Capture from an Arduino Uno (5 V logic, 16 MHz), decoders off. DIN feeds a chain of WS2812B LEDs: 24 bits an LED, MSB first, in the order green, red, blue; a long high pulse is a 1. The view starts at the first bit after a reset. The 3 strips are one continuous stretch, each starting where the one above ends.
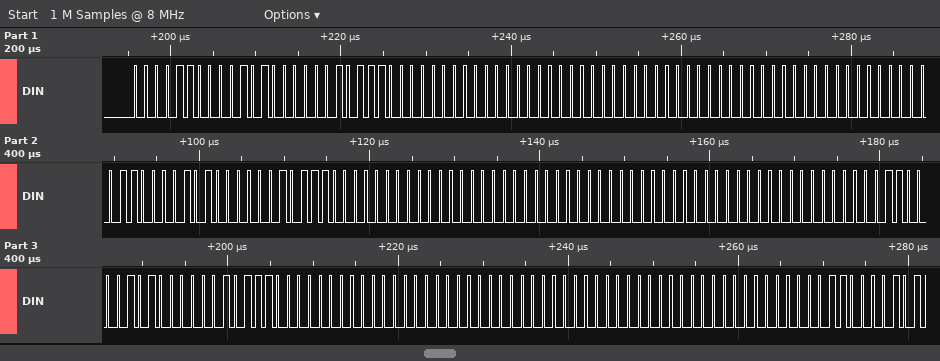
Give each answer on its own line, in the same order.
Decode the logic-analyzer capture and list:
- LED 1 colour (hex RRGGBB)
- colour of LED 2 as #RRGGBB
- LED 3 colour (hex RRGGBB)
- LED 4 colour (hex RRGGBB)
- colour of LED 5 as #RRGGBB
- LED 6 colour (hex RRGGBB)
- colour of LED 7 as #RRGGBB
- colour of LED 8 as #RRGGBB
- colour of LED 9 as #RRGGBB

#280C17
#000000
#000000
#280C17
#000000
#000000
#280C17
#000000
#000000
